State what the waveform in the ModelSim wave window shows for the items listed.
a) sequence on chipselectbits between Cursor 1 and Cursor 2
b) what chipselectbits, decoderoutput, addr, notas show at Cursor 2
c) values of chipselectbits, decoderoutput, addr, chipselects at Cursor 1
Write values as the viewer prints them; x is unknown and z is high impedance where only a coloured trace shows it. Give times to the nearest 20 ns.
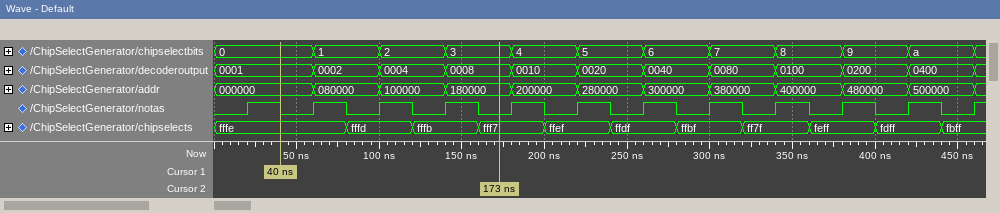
0, 1, 2, 3
chipselectbits=3, decoderoutput=0008, addr=180000, notas=0
chipselectbits=0, decoderoutput=0001, addr=000000, chipselects=fffe
